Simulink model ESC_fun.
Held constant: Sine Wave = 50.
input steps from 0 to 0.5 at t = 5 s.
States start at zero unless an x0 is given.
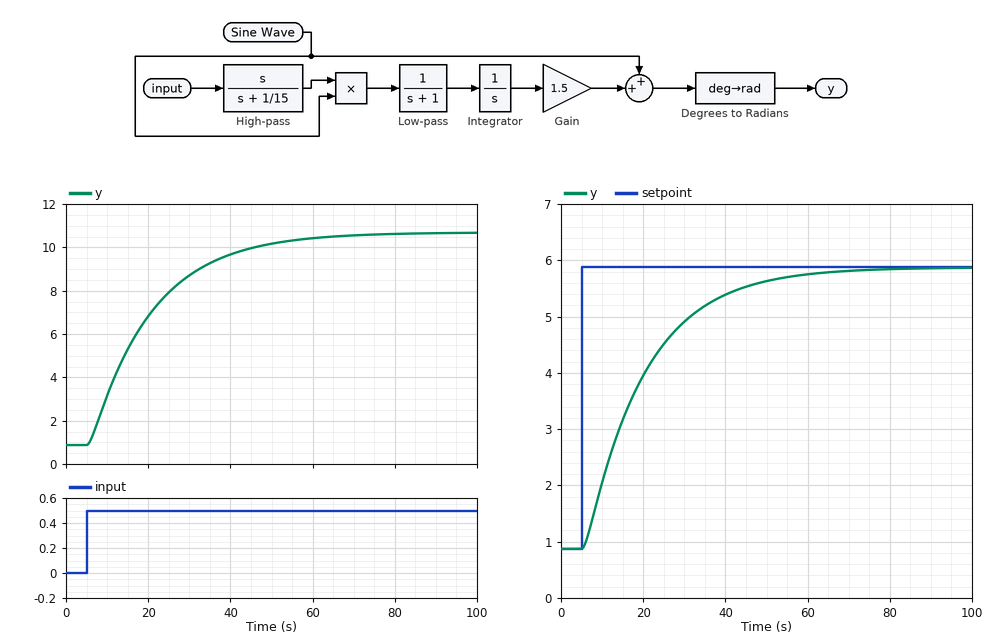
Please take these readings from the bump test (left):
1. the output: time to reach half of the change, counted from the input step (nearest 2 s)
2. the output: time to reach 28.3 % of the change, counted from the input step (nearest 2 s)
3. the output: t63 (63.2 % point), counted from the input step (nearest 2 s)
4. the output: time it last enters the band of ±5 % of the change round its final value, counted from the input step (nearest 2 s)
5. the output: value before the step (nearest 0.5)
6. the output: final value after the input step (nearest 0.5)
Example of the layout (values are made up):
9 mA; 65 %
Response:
12 s; 6 s; 16 s; 46 s; 1.0; 10.5
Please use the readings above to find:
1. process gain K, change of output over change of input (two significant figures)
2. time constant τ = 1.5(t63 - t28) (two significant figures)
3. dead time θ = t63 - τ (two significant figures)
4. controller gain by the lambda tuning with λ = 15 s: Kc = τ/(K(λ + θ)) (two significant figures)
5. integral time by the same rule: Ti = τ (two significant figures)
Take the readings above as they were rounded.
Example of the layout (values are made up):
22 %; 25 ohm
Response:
19; 15 s; 1.0 s; 0.049; 15 s
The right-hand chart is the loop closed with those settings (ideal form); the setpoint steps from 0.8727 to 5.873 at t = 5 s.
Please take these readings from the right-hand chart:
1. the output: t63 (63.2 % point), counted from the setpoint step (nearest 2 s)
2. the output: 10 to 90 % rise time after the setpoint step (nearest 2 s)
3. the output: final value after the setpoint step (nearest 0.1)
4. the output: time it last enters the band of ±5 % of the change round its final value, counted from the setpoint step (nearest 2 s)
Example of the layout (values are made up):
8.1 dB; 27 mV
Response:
16 s; 32 s; 5.9; 44 s
